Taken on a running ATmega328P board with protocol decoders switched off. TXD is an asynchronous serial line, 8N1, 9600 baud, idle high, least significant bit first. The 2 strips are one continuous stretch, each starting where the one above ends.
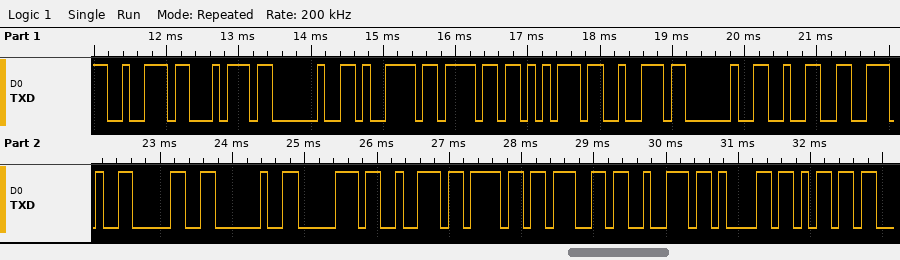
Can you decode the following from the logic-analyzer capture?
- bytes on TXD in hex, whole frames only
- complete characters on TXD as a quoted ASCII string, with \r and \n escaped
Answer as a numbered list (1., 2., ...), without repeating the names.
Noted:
1. 72 74 20 79 6F 75 72 20 32 2E 30 20 70 72 6F 67 72 61 6D
2. "rt your 2.0 program"
